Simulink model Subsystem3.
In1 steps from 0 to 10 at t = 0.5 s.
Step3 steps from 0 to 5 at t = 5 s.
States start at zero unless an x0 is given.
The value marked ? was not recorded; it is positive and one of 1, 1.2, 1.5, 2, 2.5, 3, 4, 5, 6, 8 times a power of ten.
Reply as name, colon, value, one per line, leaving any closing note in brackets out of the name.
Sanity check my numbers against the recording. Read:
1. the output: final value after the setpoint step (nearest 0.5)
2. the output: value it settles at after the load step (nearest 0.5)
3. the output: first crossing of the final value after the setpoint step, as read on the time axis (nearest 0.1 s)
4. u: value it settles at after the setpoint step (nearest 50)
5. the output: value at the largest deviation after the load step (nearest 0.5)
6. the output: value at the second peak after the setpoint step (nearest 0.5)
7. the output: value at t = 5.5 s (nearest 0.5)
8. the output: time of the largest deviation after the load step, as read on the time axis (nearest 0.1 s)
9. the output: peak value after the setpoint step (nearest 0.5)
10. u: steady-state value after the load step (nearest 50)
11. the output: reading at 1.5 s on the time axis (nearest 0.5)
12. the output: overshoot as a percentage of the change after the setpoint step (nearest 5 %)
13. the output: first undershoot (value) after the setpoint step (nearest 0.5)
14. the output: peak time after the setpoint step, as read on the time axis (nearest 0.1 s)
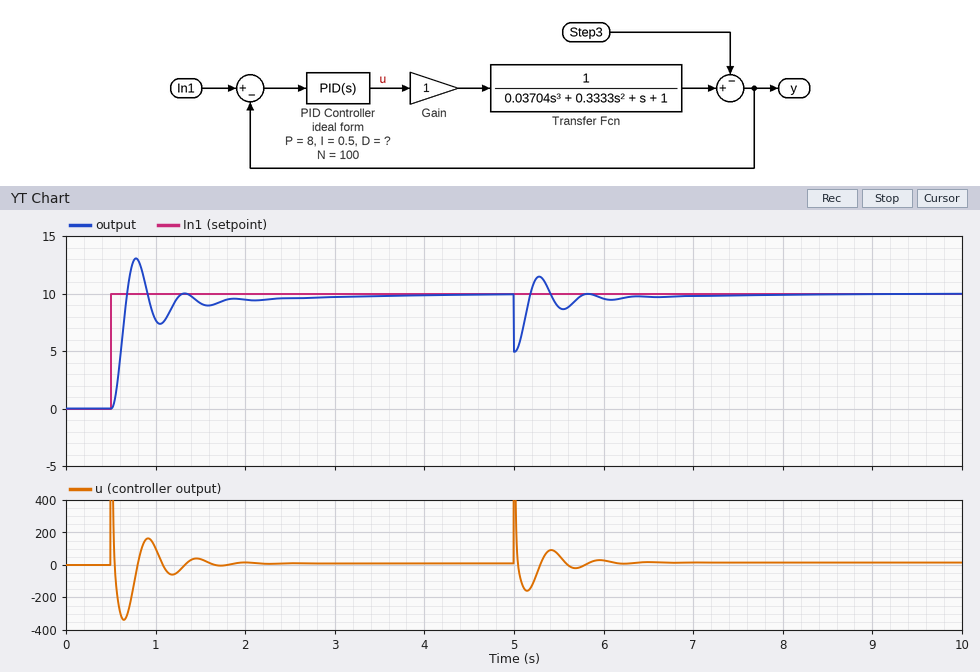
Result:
the output: final value after the setpoint step: 10.0
the output: value it settles at after the load step: 10.0
the output: first crossing of the final value after the setpoint step, as read on the time axis: 0.7 s
u: value it settles at after the setpoint step: 0
the output: value at the largest deviation after the load step: 5.0
the output: value at the second peak after the setpoint step: 10.0
the output: value at t = 5.5 s: 9.0
the output: time of the largest deviation after the load step, as read on the time axis: 5.0 s
the output: peak value after the setpoint step: 13.0
u: steady-state value after the load step: 0
the output: reading at 1.5 s on the time axis: 9.0
the output: overshoot as a percentage of the change after the setpoint step: 30 %
the output: first undershoot (value) after the setpoint step: 7.5
the output: peak time after the setpoint step, as read on the time axis: 0.8 s
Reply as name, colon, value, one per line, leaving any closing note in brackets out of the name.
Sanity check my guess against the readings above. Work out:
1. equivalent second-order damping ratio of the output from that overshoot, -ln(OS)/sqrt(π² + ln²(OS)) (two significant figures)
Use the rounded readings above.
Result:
equivalent second-order damping ratio of the output from that overshoot, -ln(OS)/sqrt(π² + ln²(OS)): 0.36
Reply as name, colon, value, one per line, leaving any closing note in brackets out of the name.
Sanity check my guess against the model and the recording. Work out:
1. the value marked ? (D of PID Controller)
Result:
the value marked ?: 0.6
